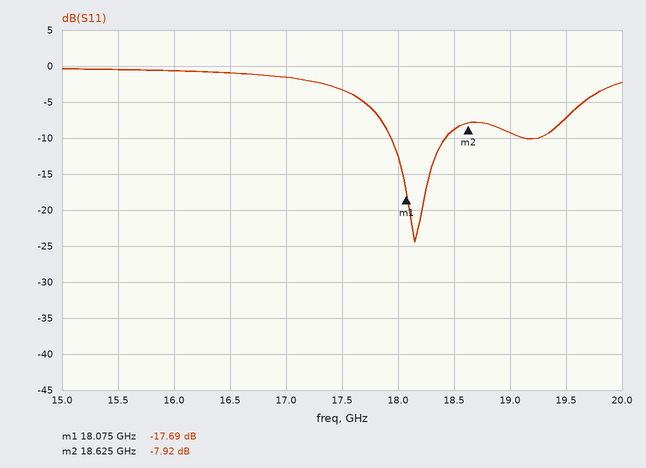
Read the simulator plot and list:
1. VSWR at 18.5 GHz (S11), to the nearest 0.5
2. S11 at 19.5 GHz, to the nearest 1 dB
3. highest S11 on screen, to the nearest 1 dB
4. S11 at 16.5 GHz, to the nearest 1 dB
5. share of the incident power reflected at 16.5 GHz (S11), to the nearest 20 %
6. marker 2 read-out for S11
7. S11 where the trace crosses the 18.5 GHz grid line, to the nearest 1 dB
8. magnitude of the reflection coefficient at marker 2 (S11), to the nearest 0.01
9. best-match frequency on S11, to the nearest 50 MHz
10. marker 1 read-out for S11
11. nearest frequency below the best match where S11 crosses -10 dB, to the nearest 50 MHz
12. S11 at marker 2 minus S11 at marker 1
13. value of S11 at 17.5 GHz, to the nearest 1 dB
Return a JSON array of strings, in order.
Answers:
["2.0", "-7 dB", "0 dB", "-1 dB", "80 %", "-7.92 dB", "-9 dB", "0.40", "18.15 GHz", "-17.69 dB", "17.95 GHz", "9.77 dB", "-3 dB"]
